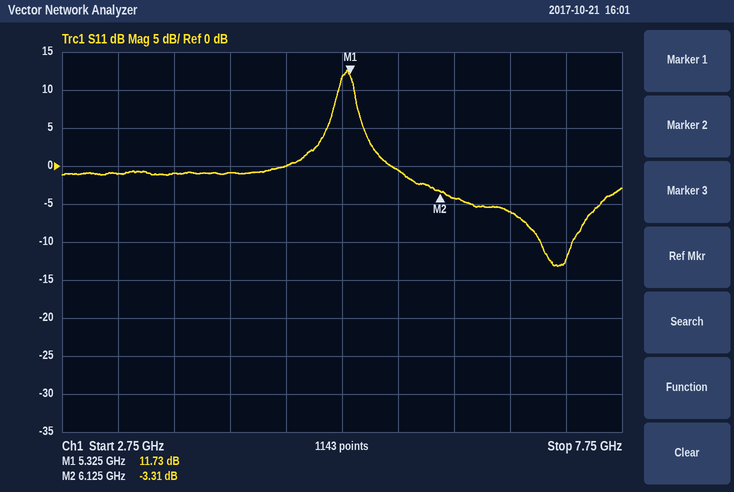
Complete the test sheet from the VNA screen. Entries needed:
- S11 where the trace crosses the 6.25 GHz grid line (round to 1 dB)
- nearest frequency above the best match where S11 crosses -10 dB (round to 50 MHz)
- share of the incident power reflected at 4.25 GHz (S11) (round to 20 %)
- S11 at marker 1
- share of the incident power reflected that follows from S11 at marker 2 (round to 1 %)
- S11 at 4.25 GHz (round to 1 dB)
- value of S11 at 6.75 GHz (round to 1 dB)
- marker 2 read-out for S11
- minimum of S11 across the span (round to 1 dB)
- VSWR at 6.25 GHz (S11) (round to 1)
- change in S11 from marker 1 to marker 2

-4 dB
7.30 GHz
80 %
11.73 dB
47 %
-1 dB
-6 dB
-3.31 dB
-13 dB
4
-15.04 dB
